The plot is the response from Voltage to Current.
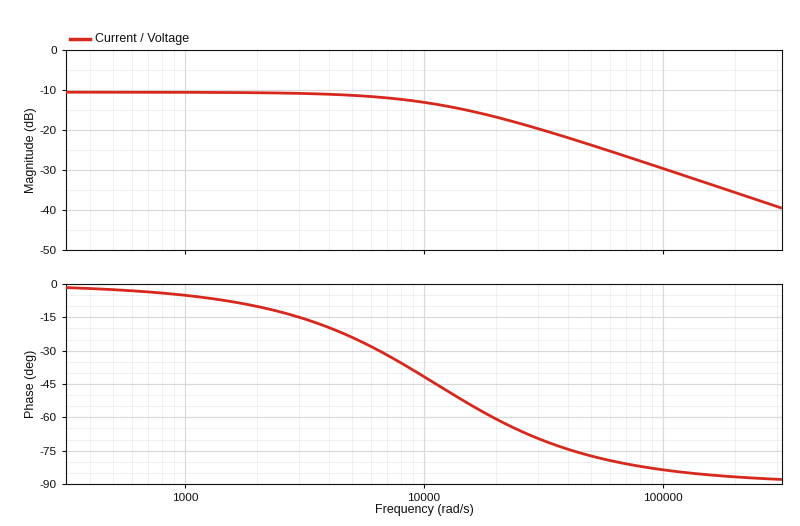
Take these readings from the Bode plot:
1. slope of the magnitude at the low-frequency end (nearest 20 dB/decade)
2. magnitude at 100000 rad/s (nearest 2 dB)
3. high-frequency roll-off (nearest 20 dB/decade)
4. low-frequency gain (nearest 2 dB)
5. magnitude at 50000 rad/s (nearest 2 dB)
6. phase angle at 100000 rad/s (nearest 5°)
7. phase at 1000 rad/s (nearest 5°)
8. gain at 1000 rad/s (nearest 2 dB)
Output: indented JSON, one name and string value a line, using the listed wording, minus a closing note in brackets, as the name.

{
  "slope of the magnitude at the low-frequency end": "0 dB/decade",
  "magnitude at 100000 rad/s": "-30 dB",
  "high-frequency roll-off": "-20 dB/decade",
  "low-frequency gain": "-10 dB",
  "magnitude at 50000 rad/s": "-24 dB",
  "phase angle at 100000 rad/s": "-85°",
  "phase at 1000 rad/s": "-5°",
  "gain at 1000 rad/s": "-10 dB"
}
